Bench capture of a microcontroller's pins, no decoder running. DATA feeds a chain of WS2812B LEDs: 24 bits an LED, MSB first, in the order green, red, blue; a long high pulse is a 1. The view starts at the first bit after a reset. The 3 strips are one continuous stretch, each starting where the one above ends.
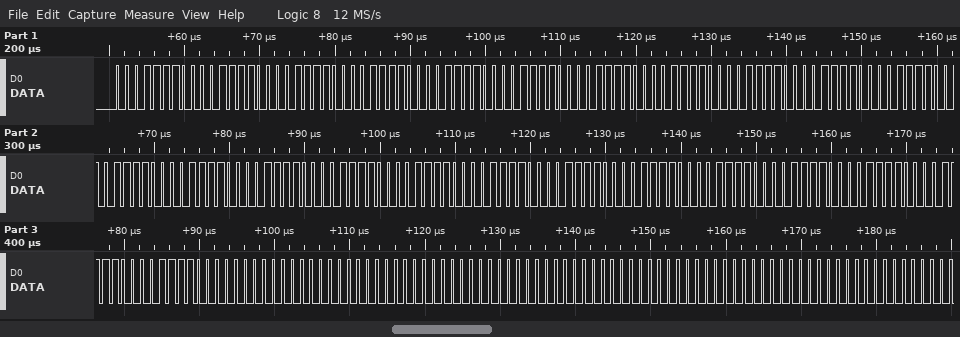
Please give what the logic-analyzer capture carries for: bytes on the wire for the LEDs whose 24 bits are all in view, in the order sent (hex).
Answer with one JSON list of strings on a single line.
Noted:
["1E 1E 1E 1E 1E 1E 1E 1E 1E 1E 1E 1E 1E 1E 1E 1E 1E 1E 1E 1E 1E 1E 1E 1E 00 00 00 00 00 00 00 00 00"]
